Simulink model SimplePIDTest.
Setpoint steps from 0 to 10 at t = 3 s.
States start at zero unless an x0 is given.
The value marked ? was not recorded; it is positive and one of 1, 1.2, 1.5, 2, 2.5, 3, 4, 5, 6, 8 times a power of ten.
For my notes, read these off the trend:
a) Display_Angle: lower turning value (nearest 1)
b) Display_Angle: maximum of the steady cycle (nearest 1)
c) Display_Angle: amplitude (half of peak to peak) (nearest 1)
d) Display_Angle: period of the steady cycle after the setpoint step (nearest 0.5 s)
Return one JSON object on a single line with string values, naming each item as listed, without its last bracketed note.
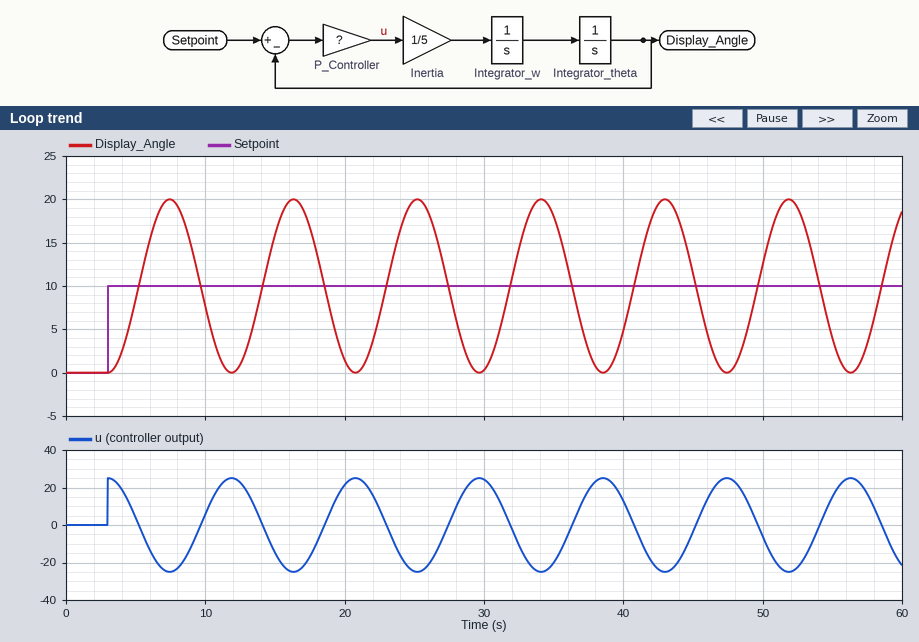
{"Display_Angle: lower turning value": "0", "Display_Angle: maximum of the steady cycle": "20", "Display_Angle: amplitude (half of peak to peak)": "10", "Display_Angle: period of the steady cycle after the setpoint step": "9.0 s"}
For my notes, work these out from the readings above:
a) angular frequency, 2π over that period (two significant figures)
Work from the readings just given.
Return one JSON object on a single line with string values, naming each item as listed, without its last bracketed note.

{"angular frequency, 2π over that period": "0.70 rad/s"}
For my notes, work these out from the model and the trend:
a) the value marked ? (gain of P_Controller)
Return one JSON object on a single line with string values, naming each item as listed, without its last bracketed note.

{"the value marked ?": "2.5"}
